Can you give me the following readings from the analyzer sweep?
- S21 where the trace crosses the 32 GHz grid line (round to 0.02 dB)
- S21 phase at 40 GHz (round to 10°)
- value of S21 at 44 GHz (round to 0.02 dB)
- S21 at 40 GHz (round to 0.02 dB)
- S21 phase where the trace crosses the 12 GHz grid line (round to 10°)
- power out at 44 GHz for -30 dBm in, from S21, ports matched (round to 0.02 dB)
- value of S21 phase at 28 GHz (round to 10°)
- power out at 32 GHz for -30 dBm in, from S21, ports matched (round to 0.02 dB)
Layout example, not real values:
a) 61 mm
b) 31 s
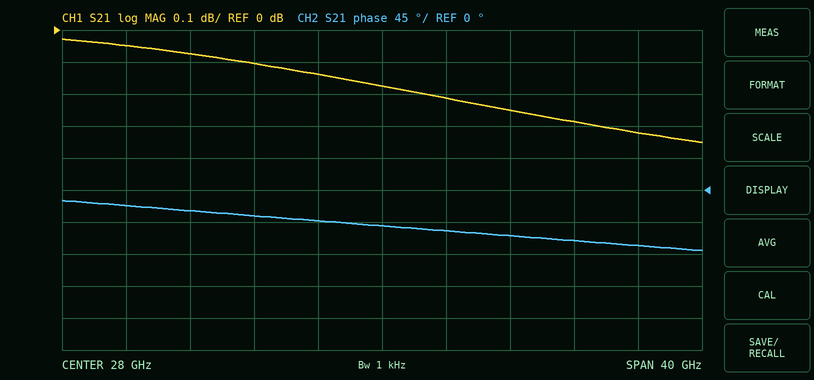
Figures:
a) -0.22 dB
b) -70°
c) -0.32 dB
d) -0.28 dB
e) -20°
f) -30.32 dBm
g) -50°
h) -30.22 dBm
